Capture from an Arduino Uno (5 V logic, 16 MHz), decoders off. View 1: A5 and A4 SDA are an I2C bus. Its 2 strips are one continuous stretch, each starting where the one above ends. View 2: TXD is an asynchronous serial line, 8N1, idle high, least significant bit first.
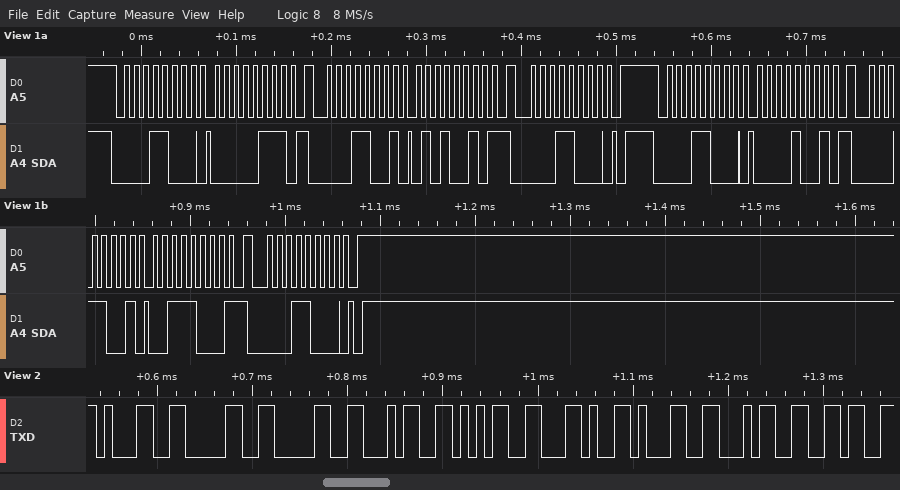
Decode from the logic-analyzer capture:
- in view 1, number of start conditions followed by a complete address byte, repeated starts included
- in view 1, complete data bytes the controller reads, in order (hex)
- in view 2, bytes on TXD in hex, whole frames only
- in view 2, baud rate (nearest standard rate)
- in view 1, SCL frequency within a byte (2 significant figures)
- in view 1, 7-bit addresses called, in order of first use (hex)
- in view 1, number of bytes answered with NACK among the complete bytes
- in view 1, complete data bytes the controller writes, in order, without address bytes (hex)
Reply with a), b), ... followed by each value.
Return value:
a) 6
b) 52 38
c) 31 30 30 34 35 2C 31 34 36
d) 115200 baud
e) 100 kHz
f) 0x0C
g) 2
h) 07 09
